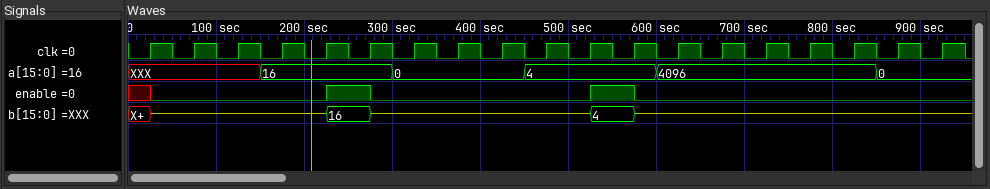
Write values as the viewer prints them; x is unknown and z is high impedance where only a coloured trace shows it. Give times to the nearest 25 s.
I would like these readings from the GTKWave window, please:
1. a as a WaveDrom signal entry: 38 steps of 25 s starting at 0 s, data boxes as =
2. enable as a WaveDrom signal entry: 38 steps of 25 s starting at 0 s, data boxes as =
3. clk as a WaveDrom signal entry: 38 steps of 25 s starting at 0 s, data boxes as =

{name: 'a', wave: 'x.....=.....=.....=.....=.........=...', data: '16 0 4 4096 0'}
{name: 'enable', wave: 'x0.......1.0.........1.0..............'}
{name: 'clk', wave: '01010101010101010101010101010101010101'}
